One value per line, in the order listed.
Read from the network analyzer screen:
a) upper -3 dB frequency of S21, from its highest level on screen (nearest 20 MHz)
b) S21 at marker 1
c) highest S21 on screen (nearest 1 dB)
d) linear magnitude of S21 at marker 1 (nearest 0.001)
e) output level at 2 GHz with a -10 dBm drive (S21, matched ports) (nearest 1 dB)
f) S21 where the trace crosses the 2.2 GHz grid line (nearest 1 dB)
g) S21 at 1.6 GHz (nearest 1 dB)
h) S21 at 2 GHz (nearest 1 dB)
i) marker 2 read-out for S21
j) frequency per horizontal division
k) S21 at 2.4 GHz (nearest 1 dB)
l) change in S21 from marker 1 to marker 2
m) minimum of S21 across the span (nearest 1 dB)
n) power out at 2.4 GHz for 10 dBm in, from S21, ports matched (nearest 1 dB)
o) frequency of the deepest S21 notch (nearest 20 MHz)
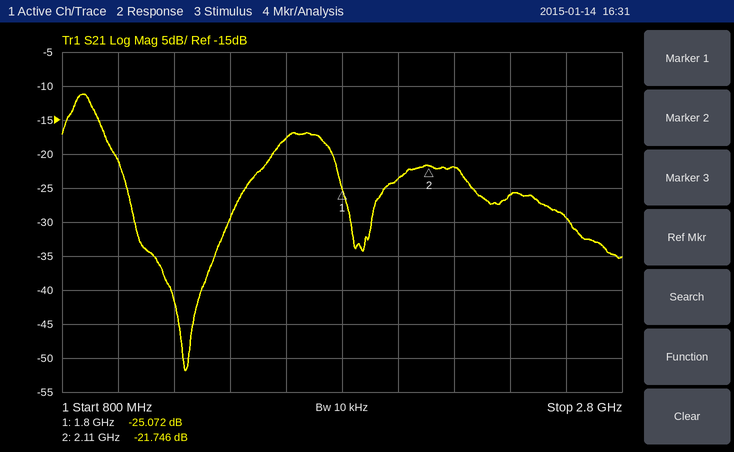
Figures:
920 MHz
-25.072 dB
-11 dB
0.056
-34 dBm
-22 dB
-18 dB
-24 dB
-21.746 dB
200 MHz
-26 dB
3.326 dB
-52 dB
-16 dBm
1.24 GHz
